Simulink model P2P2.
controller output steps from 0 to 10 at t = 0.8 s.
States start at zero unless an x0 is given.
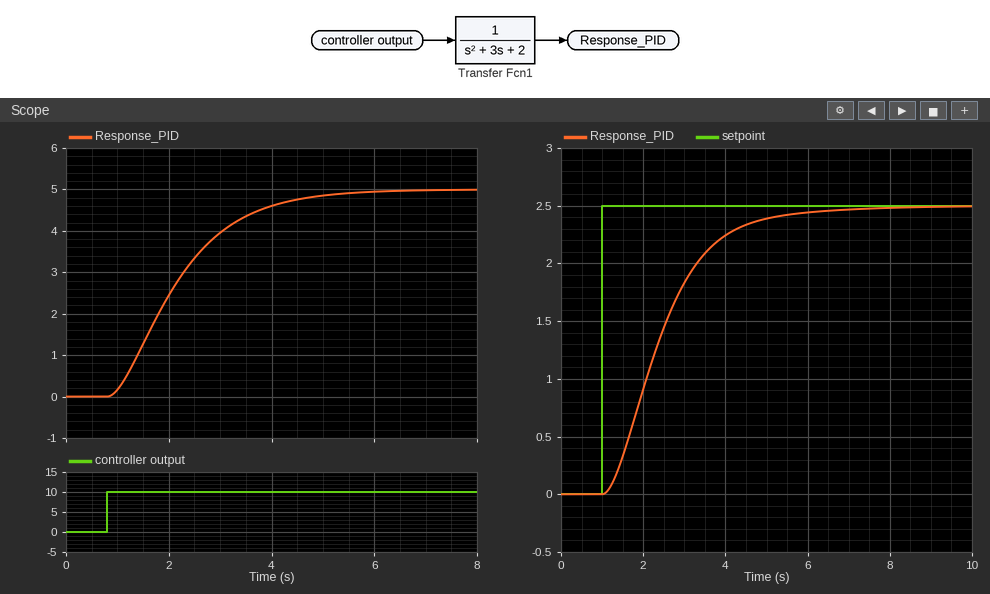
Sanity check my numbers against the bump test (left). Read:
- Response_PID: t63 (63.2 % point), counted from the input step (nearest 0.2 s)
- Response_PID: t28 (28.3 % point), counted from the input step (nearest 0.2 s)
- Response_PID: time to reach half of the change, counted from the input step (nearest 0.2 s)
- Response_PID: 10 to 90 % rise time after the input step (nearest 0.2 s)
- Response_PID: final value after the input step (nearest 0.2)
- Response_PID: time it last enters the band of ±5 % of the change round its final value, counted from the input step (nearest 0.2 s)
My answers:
1.6 s
0.8 s
1.2 s
2.6 s
5.0
3.6 s
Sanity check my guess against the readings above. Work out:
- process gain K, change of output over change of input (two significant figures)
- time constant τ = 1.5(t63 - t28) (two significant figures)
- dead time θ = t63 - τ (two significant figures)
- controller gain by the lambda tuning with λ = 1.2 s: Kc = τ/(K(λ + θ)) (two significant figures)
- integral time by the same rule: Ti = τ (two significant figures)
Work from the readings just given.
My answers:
0.50
1.2 s
0.40 s
1.5
1.2 s
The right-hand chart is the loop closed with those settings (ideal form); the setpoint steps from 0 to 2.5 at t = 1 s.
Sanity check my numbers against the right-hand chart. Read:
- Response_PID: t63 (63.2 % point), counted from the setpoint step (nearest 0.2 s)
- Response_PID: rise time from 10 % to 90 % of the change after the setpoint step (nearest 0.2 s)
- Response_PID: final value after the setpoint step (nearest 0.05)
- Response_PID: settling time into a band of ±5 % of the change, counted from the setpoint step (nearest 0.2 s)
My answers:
1.6 s
2.6 s
2.50
3.8 s
